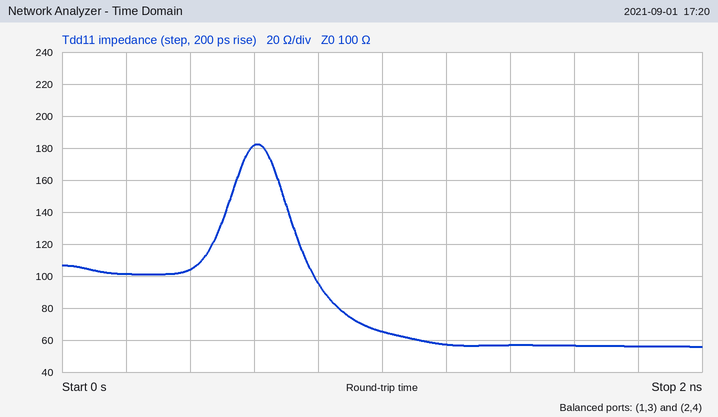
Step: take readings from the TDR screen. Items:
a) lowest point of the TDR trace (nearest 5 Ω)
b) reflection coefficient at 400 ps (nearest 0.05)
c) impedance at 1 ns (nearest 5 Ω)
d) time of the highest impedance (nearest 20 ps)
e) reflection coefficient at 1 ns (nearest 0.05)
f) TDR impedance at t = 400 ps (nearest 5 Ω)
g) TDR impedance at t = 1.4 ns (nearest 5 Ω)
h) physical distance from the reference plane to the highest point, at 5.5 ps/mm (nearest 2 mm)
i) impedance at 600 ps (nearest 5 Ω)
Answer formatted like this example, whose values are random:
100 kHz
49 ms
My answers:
55 Ω
0.00
65 Ω
620 ps
-0.20
105 Ω
55 Ω
56 mm
180 Ω
